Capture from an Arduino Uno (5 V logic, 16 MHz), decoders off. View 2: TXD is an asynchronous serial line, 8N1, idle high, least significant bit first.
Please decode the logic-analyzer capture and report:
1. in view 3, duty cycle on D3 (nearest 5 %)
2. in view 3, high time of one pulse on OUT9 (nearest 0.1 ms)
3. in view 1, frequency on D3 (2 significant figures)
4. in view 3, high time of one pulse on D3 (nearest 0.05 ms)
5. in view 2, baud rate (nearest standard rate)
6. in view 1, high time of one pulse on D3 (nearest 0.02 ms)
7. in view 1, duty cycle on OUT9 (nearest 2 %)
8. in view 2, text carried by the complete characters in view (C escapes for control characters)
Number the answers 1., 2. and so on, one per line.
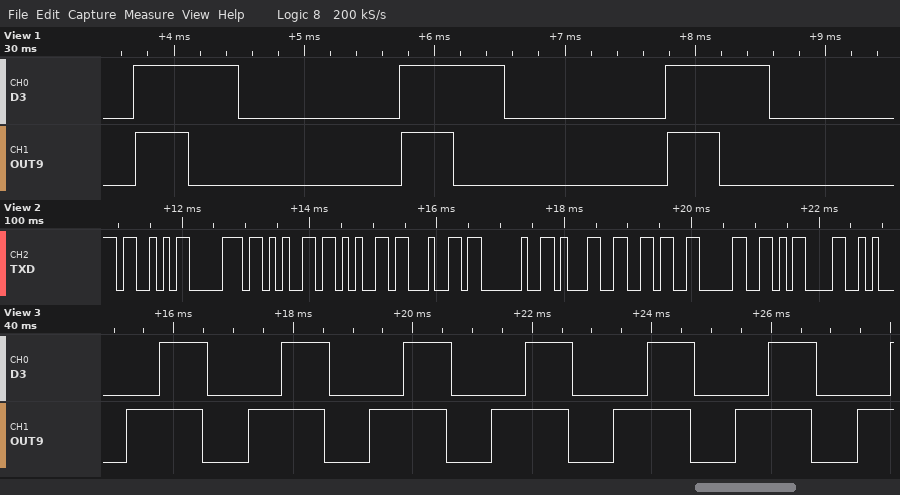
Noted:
1. 40 %
2. 1.3 ms
3. 490 Hz
4. 0.80 ms
5. 9600 baud
6. 0.80 ms
7. 20 %
8. "Speed 160\r"
